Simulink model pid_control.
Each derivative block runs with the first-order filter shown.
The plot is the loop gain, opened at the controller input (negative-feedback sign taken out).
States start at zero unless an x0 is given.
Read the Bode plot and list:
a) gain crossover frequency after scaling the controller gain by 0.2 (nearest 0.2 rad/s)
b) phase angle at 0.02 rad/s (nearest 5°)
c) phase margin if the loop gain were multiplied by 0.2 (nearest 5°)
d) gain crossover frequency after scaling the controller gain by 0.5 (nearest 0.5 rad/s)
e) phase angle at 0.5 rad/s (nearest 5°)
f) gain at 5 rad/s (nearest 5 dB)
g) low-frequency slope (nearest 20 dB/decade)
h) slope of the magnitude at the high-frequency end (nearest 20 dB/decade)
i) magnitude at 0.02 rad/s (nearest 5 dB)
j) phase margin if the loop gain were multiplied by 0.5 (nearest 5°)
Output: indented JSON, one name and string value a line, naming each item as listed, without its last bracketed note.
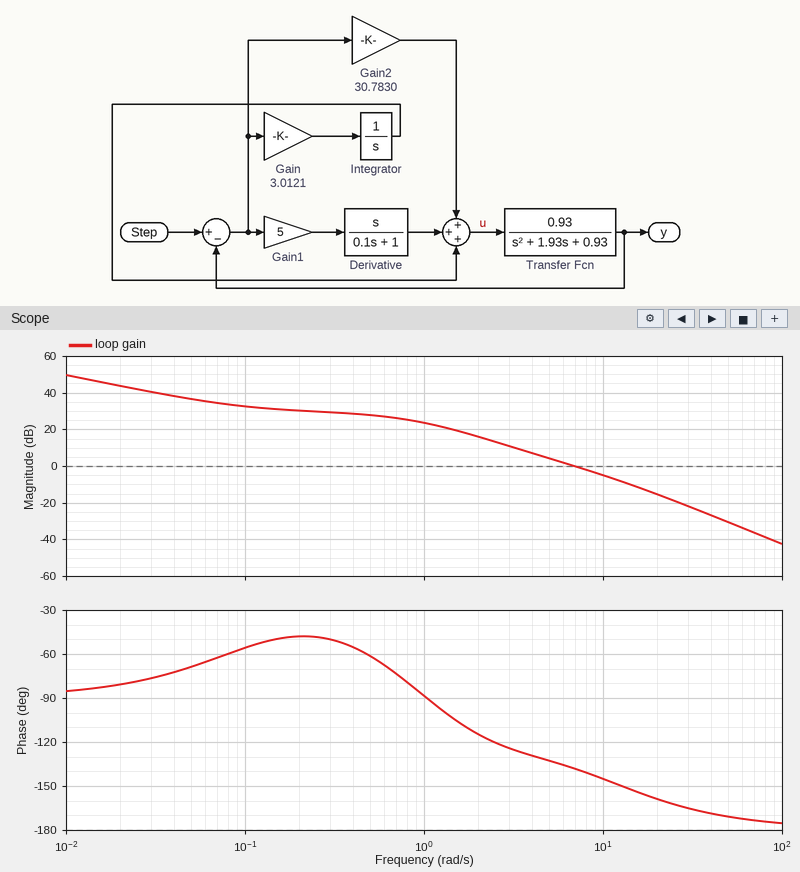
{
  "gain crossover frequency after scaling the controller gain by 0.2": "2.4 rad/s",
  "phase angle at 0.02 rad/s": "-80°",
  "phase margin if the loop gain were multiplied by 0.2": "60°",
  "gain crossover frequency after scaling the controller gain by 0.5": "4.5 rad/s",
  "phase angle at 0.5 rad/s": "-60°",
  "gain at 5 rad/s": "5 dB",
  "low-frequency slope": "-20 dB/decade",
  "slope of the magnitude at the high-frequency end": "-40 dB/decade",
  "magnitude at 0.02 rad/s": "45 dB",
  "phase margin if the loop gain were multiplied by 0.5": "50°"
}
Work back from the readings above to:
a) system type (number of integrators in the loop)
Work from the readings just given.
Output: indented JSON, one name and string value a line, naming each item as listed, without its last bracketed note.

{
  "system type": "1"
}
